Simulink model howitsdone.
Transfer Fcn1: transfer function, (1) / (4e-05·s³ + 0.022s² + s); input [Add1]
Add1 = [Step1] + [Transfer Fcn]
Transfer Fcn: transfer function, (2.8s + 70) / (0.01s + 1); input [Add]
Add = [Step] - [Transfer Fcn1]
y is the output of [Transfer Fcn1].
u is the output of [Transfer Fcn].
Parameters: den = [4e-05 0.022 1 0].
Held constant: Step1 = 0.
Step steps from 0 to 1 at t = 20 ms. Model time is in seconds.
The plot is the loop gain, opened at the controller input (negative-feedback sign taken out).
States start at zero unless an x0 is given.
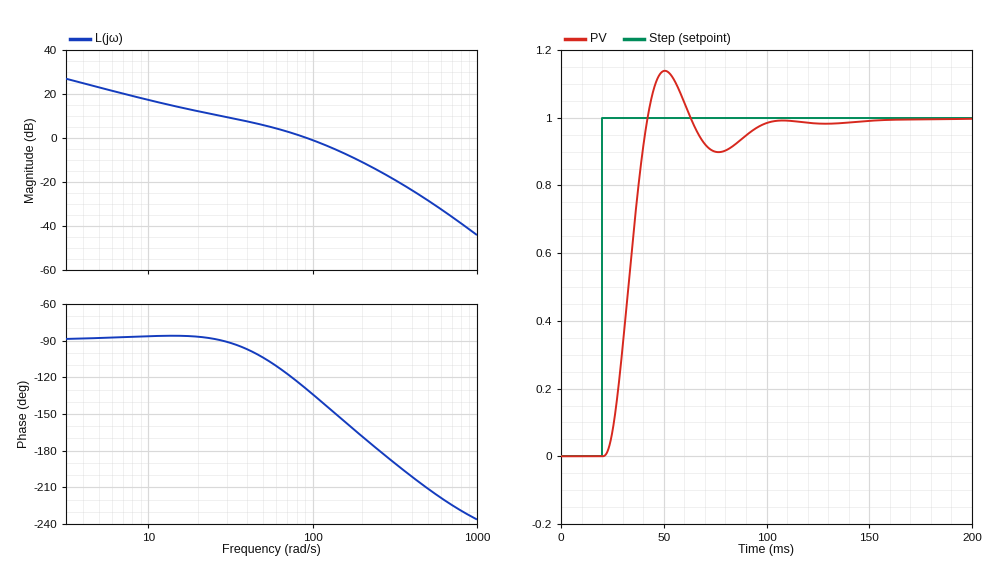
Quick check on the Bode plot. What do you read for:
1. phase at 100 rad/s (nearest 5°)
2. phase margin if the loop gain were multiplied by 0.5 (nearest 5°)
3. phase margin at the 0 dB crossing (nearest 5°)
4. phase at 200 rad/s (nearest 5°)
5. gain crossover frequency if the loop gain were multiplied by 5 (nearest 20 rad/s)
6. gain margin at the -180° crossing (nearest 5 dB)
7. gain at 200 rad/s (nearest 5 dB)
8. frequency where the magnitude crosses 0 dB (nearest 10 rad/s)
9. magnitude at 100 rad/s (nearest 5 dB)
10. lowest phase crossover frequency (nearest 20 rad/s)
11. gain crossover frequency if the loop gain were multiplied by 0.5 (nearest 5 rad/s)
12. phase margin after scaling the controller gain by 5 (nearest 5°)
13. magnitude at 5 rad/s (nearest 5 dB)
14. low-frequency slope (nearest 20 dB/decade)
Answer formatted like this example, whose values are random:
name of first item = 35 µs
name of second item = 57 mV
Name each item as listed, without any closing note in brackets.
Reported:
phase at 100 rad/s = -135°
phase margin if the loop gain were multiplied by 0.5 = 75°
phase margin at the 0 dB crossing = 50°
phase at 200 rad/s = -170°
gain crossover frequency if the loop gain were multiplied by 5 = 240 rad/s
gain margin at the -180° crossing = 15 dB
gain at 200 rad/s = -10 dB
frequency where the magnitude crosses 0 dB = 90 rad/s
magnitude at 100 rad/s = 0 dB
lowest phase crossover frequency = 260 rad/s
gain crossover frequency if the loop gain were multiplied by 0.5 = 50 rad/s
phase margin after scaling the controller gain by 5 = 5°
magnitude at 5 rad/s = 25 dB
low-frequency slope = -20 dB/decade
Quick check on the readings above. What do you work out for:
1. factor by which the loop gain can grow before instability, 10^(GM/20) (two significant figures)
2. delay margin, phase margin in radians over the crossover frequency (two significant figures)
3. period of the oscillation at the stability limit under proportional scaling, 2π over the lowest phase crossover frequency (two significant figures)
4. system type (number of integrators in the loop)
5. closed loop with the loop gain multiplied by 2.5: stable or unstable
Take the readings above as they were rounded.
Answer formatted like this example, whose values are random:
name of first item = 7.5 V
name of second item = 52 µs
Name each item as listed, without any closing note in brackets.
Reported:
factor by which the loop gain can grow before instability, 10^(GM/20) = 5.6
delay margin, phase margin in radians over the crossover frequency = 0.0097 s
period of the oscillation at the stability limit under proportional scaling, 2π over the lowest phase crossover frequency = 0.024 s
system type = 1
closed loop with the loop gain multiplied by 2.5: stable or unstable = stable
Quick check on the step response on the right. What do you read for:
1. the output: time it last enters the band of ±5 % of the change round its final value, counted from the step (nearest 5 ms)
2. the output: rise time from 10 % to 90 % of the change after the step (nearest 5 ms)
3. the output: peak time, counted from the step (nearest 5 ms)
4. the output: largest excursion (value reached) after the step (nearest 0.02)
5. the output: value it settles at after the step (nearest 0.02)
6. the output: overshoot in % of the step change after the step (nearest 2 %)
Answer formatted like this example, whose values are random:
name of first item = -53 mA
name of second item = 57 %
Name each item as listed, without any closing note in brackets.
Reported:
the output: time it last enters the band of ±5 % of the change round its final value, counted from the step = 70 ms
the output: rise time from 10 % to 90 % of the change after the step = 15 ms
the output: peak time, counted from the step = 30 ms
the output: largest excursion (value reached) after the step = 1.14
the output: value it settles at after the step = 1.00
the output: overshoot in % of the step change after the step = 14 %
